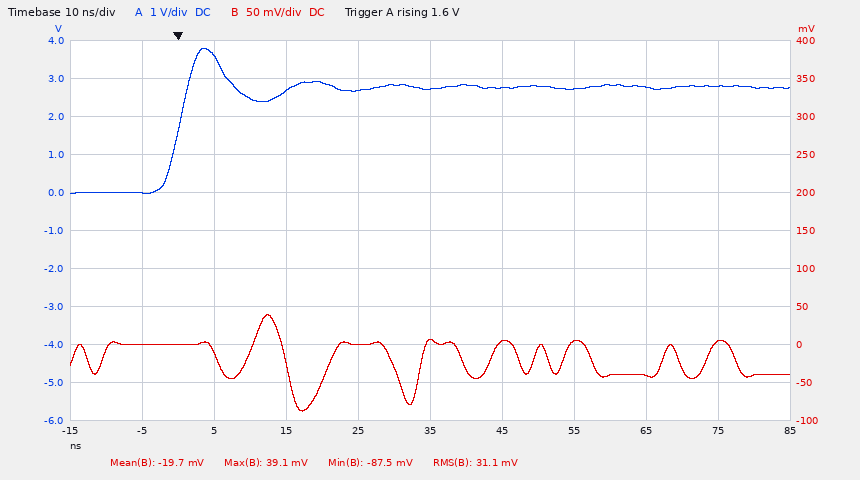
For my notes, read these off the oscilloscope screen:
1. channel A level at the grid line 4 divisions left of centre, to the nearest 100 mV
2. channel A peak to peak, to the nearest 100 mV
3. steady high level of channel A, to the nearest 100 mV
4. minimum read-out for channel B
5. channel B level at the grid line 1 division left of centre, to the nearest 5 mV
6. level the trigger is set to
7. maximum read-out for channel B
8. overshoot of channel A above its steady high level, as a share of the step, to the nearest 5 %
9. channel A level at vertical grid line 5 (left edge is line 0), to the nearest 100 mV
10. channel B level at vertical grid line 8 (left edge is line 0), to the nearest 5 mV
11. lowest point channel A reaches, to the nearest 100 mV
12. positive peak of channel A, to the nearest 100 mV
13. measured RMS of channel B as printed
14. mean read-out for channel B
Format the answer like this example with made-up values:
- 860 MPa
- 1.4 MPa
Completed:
- 0.0 V
- 3.8 V
- 2.8 V
- -87.5 mV
- 0 mV
- 1.6 V
- 39.1 mV
- 35 %
- 2.7 V
- -40 mV
- 0.0 V
- 3.8 V
- 31.1 mV
- -19.7 mV
